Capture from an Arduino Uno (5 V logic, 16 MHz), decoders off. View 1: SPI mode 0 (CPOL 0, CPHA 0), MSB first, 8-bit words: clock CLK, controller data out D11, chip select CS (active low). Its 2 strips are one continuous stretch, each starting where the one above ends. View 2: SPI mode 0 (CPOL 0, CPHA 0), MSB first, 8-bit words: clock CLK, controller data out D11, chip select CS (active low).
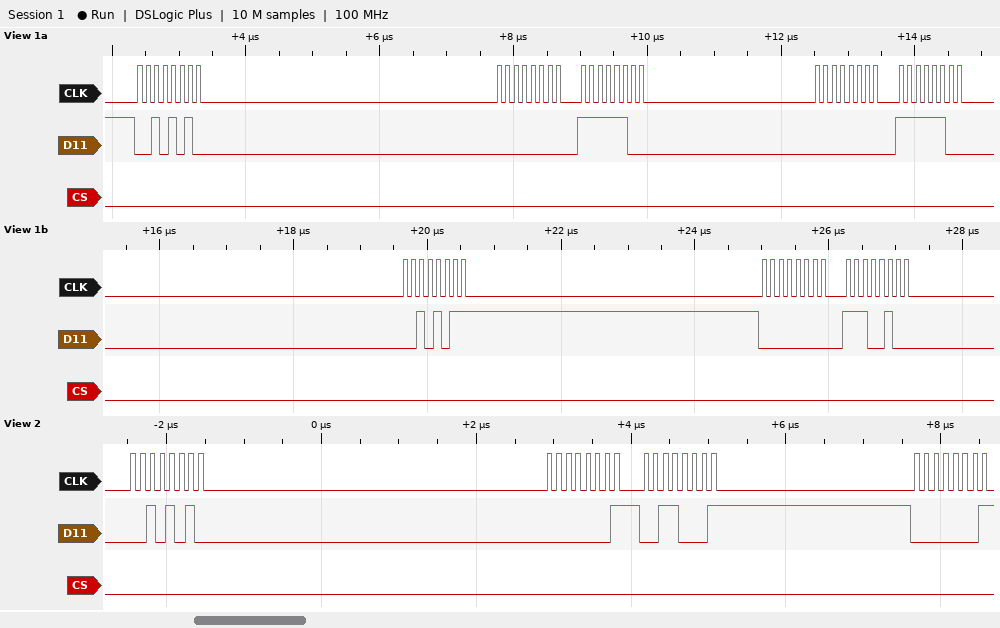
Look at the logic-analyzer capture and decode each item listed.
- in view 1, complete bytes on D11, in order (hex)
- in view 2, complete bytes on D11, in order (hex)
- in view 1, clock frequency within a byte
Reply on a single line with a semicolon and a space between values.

2A 00 FC 00 FC 2B 00 E4; 2A 01 31 01; 8 MHz
